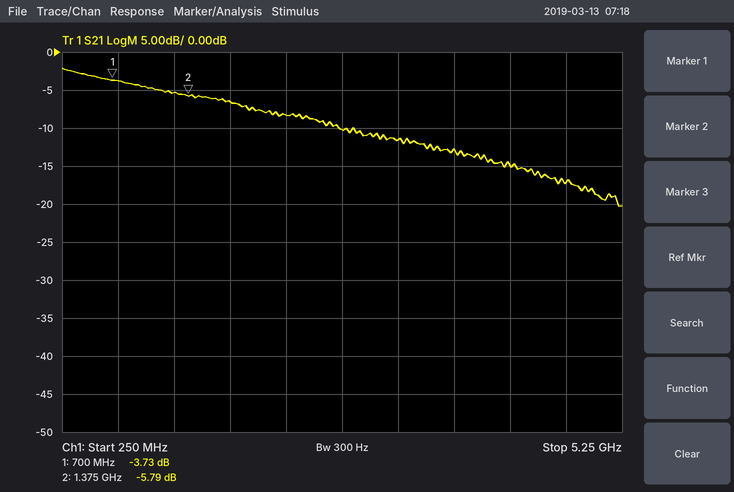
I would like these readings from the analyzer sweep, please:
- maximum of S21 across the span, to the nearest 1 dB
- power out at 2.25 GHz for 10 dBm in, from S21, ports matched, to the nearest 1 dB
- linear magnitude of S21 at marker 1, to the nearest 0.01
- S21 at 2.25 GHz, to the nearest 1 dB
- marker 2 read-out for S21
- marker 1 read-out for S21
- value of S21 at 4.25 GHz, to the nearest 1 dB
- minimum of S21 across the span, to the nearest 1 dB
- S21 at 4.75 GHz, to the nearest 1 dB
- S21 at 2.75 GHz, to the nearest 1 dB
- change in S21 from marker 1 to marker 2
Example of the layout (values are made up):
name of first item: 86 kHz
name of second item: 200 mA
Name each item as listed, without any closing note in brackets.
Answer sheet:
maximum of S21 across the span, to the nearest 1 dB: -2 dB
power out at 2.25 GHz for 10 dBm in, from S21, ports matched, to the nearest 1 dB: 2 dBm
linear magnitude of S21 at marker 1, to the nearest 0.01: 0.65
S21 at 2.25 GHz, to the nearest 1 dB: -8 dB
marker 2 read-out for S21: -5.79 dB
marker 1 read-out for S21: -3.73 dB
value of S21 at 4.25 GHz, to the nearest 1 dB: -15 dB
minimum of S21 across the span, to the nearest 1 dB: -20 dB
S21 at 4.75 GHz, to the nearest 1 dB: -17 dB
S21 at 2.75 GHz, to the nearest 1 dB: -10 dB
change in S21 from marker 1 to marker 2: -2.06 dB
